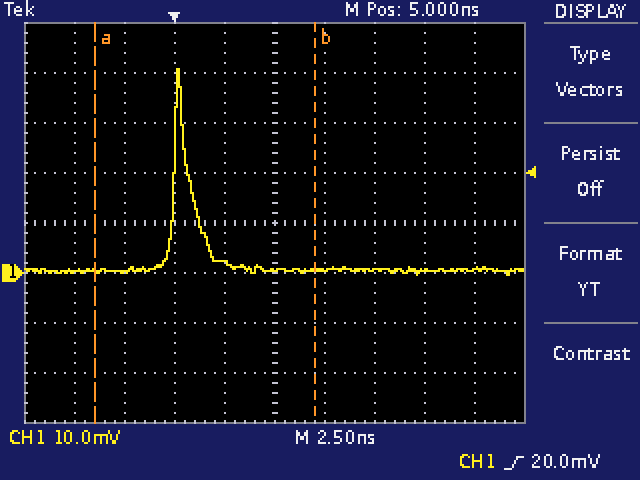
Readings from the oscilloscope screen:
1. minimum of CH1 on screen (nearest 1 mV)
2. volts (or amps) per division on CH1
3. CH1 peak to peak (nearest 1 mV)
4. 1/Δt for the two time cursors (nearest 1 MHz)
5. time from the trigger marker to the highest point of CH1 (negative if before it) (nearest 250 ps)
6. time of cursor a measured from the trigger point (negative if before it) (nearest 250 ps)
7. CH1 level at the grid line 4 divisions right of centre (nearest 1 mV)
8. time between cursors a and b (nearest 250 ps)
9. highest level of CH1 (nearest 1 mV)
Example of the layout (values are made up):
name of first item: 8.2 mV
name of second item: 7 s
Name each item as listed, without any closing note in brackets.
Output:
minimum of CH1 on screen: 0 mV
volts (or amps) per division on CH1: 10 mV
CH1 peak to peak: 41 mV
1/Δt for the two time cursors: 91 MHz
time from the trigger marker to the highest point of CH1 (negative if before it): +250 ps
time of cursor a measured from the trigger point (negative if before it): -4.00 ns
CH1 level at the grid line 4 divisions right of centre: 1 mV
time between cursors a and b: 11.00 ns
highest level of CH1: 41 mV
